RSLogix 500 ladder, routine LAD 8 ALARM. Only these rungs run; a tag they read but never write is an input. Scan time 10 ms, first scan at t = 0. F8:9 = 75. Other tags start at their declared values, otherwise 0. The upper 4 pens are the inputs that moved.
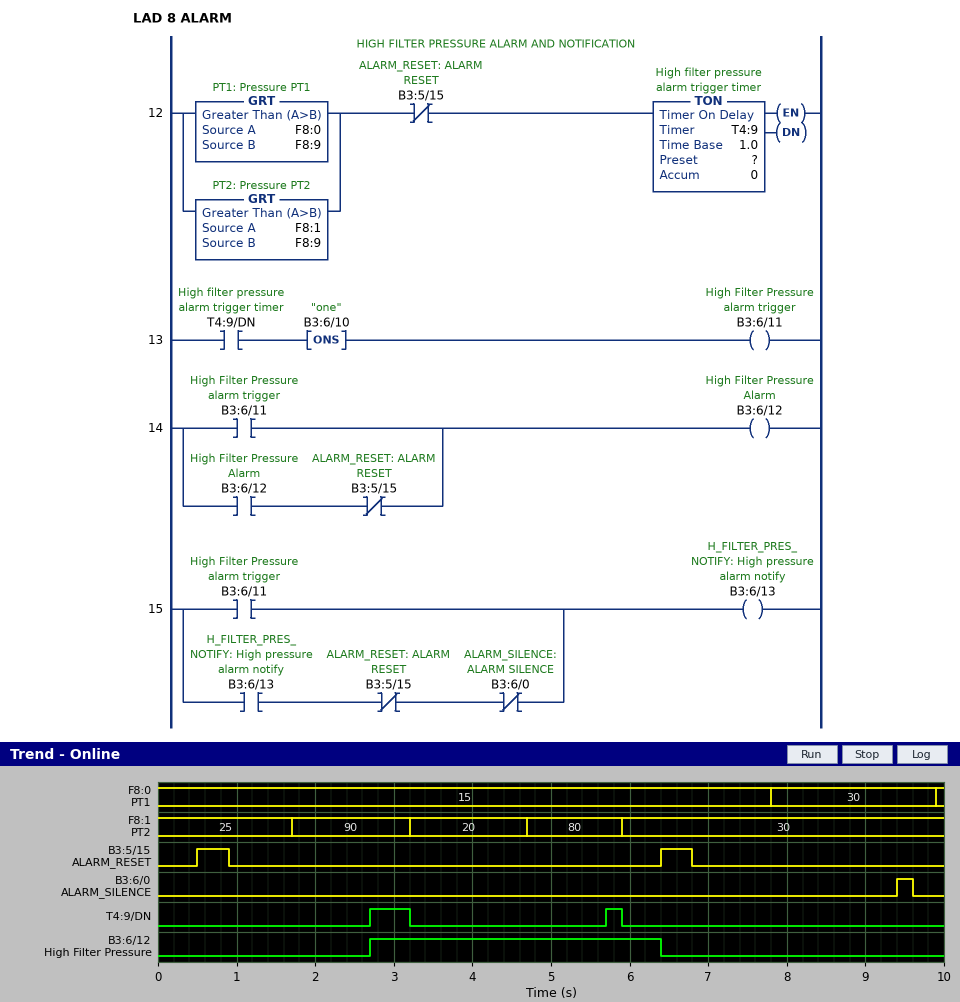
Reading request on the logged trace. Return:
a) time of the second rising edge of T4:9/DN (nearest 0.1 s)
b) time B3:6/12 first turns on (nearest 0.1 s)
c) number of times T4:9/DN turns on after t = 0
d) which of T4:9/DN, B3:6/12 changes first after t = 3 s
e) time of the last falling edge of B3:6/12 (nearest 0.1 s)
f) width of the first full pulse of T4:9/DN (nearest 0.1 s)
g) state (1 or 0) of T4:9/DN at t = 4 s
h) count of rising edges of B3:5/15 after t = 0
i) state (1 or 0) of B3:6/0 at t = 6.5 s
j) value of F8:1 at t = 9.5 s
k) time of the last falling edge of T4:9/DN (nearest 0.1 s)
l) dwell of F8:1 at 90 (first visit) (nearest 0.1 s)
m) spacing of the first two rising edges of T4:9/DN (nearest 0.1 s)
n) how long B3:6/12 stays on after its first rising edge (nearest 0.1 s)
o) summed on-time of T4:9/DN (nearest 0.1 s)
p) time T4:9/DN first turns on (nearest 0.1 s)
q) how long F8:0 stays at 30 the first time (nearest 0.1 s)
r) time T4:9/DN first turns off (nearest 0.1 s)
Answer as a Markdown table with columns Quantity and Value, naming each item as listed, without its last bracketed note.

| Quantity | Value |
|---|---|
| time of the second rising edge of T4:9/DN | 5.7 s |
| time B3:6/12 first turns on | 2.7 s |
| number of times T4:9/DN turns on after t = 0 | 2 |
| which of T4:9/DN, B3:6/12 changes first after t = 3 s | T4:9/DN |
| time of the last falling edge of B3:6/12 | 6.4 s |
| width of the first full pulse of T4:9/DN | 0.5 s |
| state (1 or 0) of T4:9/DN at t = 4 s | 0 |
| count of rising edges of B3:5/15 after t = 0 | 2 |
| state (1 or 0) of B3:6/0 at t = 6.5 s | 0 |
| value of F8:1 at t = 9.5 s | 30 |
| time of the last falling edge of T4:9/DN | 5.9 s |
| dwell of F8:1 at 90 (first visit) | 1.5 s |
| spacing of the first two rising edges of T4:9/DN | 3.0 s |
| how long B3:6/12 stays on after its first rising edge | 3.7 s |
| summed on-time of T4:9/DN | 0.7 s |
| time T4:9/DN first turns on | 2.7 s |
| how long F8:0 stays at 30 the first time | 2.1 s |
| time T4:9/DN first turns off | 3.2 s |
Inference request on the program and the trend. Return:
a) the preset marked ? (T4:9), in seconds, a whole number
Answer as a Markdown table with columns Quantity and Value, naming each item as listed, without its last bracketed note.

| Quantity | Value |
|---|---|
| the preset marked ? (T4:9), in seconds, a whole number | 1 s |
